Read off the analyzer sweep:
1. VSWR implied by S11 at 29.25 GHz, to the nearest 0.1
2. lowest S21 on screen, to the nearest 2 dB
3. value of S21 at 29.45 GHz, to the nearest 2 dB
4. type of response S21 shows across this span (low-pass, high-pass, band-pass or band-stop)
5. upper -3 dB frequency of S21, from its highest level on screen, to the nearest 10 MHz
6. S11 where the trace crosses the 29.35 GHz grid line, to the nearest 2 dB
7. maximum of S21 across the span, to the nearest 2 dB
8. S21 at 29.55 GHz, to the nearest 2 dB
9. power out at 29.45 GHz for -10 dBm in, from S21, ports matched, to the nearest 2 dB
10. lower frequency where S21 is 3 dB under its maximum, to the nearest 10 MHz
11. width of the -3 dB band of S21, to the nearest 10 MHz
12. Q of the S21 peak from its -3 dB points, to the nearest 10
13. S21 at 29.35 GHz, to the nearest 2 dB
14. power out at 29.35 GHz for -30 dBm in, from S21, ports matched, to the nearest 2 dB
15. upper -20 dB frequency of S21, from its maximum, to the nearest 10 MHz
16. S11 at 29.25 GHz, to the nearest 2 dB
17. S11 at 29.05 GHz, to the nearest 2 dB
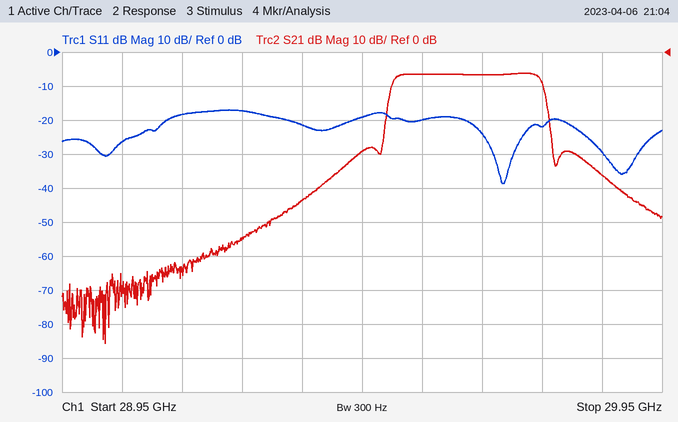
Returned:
1.3
-86 dB
-30 dB
band-pass
29.75 GHz
-22 dB
-6 dB
-6 dB
-40 dBm
29.50 GHz
250 MHz
120
-44 dB
-74 dBm
29.77 GHz
-18 dB
-26 dB
